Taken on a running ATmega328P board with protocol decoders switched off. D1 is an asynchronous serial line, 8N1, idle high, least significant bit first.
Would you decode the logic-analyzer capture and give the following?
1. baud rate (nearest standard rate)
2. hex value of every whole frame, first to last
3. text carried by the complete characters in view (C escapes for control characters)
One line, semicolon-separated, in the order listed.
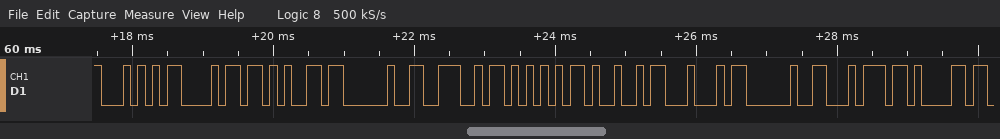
9600 baud; 0x54 0x68 0x65 0x20 0x4E 0x55 0x49 0x44 0x20 0x74 0x61; "The NUID ta"
